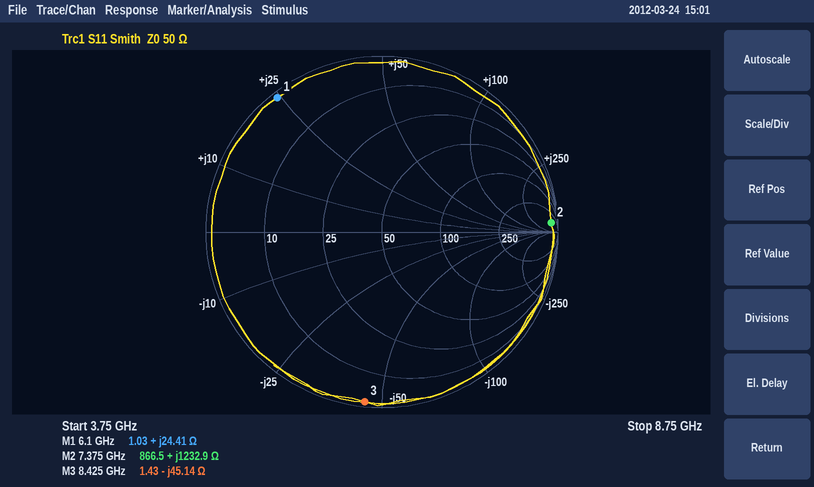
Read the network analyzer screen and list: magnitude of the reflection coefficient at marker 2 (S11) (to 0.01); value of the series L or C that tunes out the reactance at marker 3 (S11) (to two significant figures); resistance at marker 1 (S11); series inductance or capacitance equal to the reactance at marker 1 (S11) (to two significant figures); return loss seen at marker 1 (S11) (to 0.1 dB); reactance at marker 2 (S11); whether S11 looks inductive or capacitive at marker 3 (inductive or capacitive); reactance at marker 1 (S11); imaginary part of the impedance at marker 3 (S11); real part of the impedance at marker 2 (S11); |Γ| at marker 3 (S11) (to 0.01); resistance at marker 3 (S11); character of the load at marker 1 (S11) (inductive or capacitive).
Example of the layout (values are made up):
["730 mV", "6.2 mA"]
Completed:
["0.96", "850 pH", "1.03 Ω", "640 pH", "0.3 dB", "+1232.9 Ω", "capacitive", "+24.41 Ω", "-45.14 Ω", "866.5 Ω", "0.97", "1.43 Ω", "inductive"]
